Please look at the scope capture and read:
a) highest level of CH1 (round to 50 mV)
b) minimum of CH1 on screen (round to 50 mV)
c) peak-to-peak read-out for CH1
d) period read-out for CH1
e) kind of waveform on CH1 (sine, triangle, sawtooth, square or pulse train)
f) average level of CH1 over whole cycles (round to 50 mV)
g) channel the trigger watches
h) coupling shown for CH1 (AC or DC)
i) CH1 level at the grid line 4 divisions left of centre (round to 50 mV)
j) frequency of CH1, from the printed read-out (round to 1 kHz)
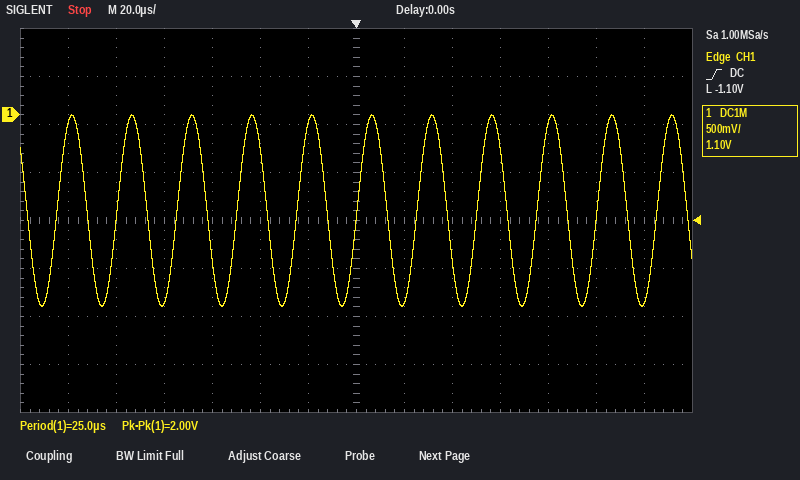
0 mV
-2.00 V
2.00 V
25.0 µs
sine
-1.00 V
CH1
DC
-1.95 V
40 kHz
